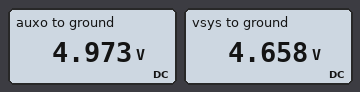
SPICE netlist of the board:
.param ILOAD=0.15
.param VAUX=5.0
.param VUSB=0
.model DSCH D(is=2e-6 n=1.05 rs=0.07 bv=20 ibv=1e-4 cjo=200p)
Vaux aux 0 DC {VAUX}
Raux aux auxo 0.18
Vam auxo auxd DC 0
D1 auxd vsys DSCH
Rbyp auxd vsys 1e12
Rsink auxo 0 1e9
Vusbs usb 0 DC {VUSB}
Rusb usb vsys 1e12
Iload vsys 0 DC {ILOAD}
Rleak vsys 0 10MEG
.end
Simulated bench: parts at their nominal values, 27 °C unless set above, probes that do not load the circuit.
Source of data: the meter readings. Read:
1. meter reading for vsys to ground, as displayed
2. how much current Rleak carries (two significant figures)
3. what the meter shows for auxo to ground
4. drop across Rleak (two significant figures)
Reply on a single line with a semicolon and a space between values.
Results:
4.658 V; 470 nA; 4.973 V; 4.7 V
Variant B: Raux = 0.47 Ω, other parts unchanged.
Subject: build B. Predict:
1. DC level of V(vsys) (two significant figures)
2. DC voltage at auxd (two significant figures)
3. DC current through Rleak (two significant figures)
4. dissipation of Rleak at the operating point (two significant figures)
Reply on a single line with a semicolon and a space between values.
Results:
4.6 V; 4.9 V; 460 nA; 2.1 µW
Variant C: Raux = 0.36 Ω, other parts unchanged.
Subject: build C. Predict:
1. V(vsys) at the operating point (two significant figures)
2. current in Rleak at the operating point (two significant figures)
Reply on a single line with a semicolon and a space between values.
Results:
4.6 V; 460 nA
